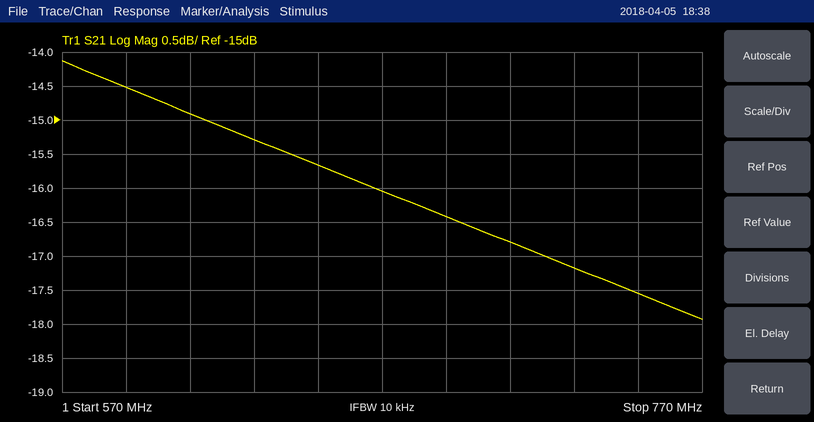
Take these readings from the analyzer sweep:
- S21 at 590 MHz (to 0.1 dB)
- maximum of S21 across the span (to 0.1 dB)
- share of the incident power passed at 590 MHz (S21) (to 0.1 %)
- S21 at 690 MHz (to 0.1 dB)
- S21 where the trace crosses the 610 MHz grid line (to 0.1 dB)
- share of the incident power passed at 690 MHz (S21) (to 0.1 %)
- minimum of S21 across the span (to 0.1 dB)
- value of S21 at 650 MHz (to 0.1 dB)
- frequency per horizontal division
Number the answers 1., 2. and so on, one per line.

1. -14.5 dB
2. -14.1 dB
3. 3.5 %
4. -16.4 dB
5. -14.9 dB
6. 2.3 %
7. -17.9 dB
8. -15.7 dB
9. 20 MHz
